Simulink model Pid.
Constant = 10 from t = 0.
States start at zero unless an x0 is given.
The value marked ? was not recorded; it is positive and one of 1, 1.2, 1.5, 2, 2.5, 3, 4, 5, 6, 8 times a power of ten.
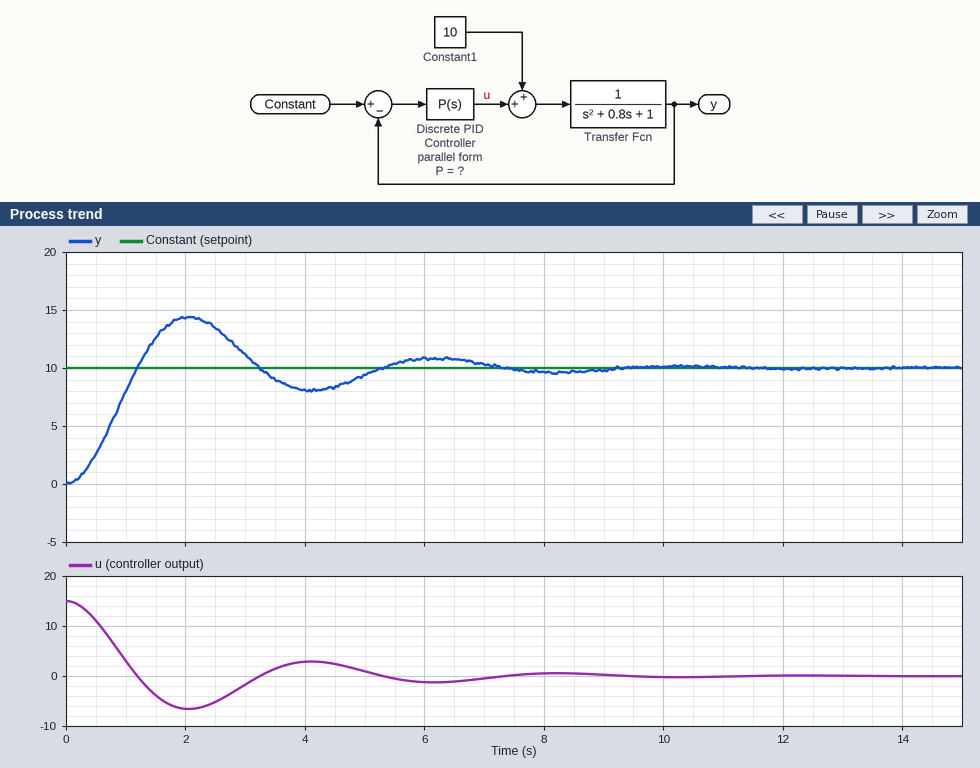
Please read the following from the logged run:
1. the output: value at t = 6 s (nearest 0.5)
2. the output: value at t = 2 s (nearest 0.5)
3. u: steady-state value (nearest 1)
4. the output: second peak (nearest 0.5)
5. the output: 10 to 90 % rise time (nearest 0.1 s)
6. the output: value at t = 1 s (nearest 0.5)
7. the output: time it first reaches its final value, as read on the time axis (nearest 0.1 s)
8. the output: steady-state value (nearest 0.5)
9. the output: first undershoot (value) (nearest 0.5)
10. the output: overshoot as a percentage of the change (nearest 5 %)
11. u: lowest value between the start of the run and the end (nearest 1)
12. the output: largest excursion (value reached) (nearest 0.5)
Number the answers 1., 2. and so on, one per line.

1. 11.0
2. 14.5
3. 0
4. 11.0
5. 0.8 s
6. 8.0
7. 1.2 s
8. 10.0
9. 8.0
10. 45 %
11. -7
12. 14.5
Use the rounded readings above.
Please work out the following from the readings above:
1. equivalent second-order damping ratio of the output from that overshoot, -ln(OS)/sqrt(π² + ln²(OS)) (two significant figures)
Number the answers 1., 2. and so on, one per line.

1. 0.25
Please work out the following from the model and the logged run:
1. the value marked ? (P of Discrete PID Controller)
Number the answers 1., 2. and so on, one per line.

1. 1.5
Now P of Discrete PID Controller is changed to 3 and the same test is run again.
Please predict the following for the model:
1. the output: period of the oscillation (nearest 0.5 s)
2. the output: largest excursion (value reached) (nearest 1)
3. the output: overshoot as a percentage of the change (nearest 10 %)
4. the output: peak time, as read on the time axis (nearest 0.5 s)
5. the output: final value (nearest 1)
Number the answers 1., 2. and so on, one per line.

1. 3.0 s
2. 15
3. 50 %
4. 1.5 s
5. 10
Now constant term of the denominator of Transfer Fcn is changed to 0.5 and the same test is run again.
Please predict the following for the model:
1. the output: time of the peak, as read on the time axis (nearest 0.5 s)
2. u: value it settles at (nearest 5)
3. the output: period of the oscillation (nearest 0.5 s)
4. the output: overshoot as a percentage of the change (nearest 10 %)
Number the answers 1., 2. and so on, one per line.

1. 2.5 s
2. -5
3. 4.5 s
4. 40 %
